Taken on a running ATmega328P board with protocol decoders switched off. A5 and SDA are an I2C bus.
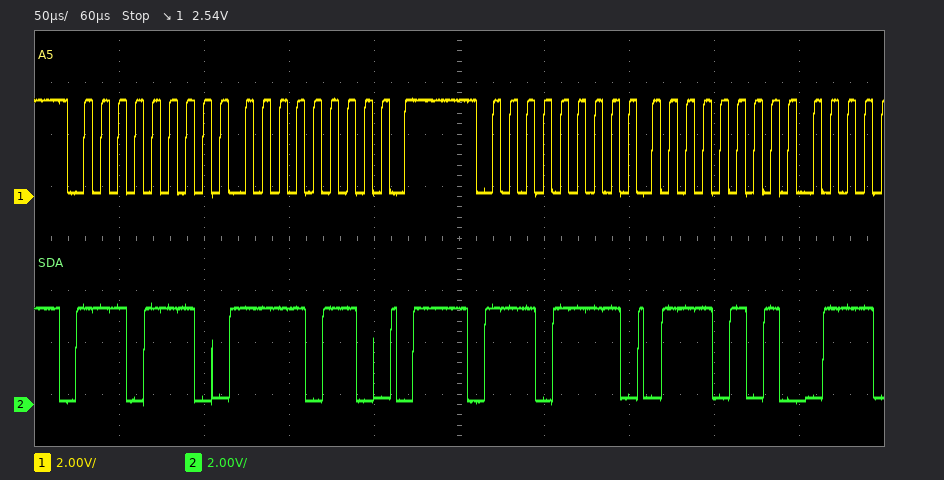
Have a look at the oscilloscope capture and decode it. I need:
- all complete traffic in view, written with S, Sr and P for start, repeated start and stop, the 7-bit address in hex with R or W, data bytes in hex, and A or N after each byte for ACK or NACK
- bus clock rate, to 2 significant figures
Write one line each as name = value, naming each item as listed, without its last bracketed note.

all complete traffic in view, written with S, Sr and P for start, repeated start and stop, the 7-bit address in hex with R or W, data bytes in hex, and A or N after each byte for ACK or NACK = S 77W A F6 A P S 77R A 75 A
bus clock rate, to 2 significant figures = 100 kHz
